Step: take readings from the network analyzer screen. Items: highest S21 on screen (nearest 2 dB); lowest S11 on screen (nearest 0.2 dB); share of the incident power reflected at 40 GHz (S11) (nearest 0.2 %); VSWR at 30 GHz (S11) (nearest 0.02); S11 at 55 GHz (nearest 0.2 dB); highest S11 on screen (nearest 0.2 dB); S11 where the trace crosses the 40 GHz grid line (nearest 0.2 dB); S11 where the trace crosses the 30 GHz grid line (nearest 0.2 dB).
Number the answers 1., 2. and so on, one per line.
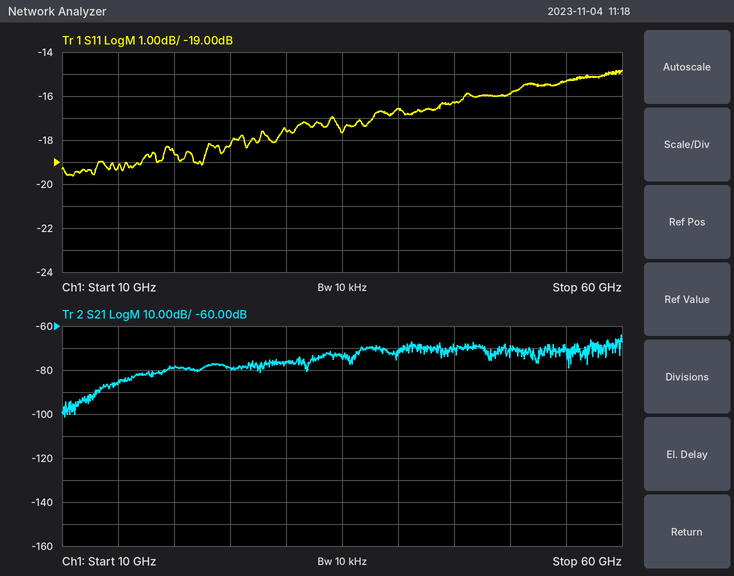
1. -64 dB
2. -19.6 dB
3. 2.2 %
4. 1.30
5. -15.4 dB
6. -14.8 dB
7. -16.6 dB
8. -17.6 dB
